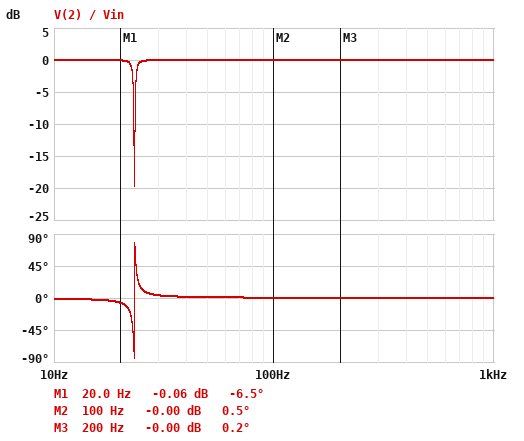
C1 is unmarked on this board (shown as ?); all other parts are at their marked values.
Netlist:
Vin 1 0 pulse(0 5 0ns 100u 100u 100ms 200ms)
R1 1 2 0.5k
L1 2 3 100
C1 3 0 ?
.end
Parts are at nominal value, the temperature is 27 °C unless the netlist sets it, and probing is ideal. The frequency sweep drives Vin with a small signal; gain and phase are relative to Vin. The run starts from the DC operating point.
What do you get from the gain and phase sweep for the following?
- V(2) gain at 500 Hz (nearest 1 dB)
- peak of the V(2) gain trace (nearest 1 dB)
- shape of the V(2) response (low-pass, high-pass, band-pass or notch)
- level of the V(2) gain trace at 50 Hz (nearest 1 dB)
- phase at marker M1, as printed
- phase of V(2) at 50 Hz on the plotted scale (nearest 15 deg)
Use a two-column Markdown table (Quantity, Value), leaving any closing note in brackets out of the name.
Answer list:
| Quantity | Value |
|---|---|
| V(2) gain at 500 Hz | 0 dB |
| peak of the V(2) gain trace | 0 dB |
| shape of the V(2) response | notch |
| level of the V(2) gain trace at 50 Hz | 0 dB |
| phase at marker M1, as printed | -6.5 deg |
| phase of V(2) at 50 Hz on the plotted scale | 0 deg |
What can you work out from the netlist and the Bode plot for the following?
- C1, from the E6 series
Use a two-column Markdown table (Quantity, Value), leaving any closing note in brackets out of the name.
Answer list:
| Quantity | Value |
|---|---|
| C1, from the E6 series | 470 nF |
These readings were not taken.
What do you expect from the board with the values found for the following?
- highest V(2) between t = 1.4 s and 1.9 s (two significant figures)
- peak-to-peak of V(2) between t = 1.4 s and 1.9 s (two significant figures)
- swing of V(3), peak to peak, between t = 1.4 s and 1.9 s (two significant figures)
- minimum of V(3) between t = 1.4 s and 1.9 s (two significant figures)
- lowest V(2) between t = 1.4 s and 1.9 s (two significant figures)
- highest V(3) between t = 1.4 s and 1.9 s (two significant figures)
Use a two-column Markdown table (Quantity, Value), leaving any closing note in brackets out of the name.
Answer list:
| Quantity | Value |
|---|---|
| highest V(2) between t = 1.4 s and 1.9 s | 5.2 V |
| peak-to-peak of V(2) between t = 1.4 s and 1.9 s | 5.3 V |
| swing of V(3), peak to peak, between t = 1.4 s and 1.9 s | 15 V |
| minimum of V(3) between t = 1.4 s and 1.9 s | -4.8 V |
| lowest V(2) between t = 1.4 s and 1.9 s | -160 mV |
| highest V(3) between t = 1.4 s and 1.9 s | 9.8 V |
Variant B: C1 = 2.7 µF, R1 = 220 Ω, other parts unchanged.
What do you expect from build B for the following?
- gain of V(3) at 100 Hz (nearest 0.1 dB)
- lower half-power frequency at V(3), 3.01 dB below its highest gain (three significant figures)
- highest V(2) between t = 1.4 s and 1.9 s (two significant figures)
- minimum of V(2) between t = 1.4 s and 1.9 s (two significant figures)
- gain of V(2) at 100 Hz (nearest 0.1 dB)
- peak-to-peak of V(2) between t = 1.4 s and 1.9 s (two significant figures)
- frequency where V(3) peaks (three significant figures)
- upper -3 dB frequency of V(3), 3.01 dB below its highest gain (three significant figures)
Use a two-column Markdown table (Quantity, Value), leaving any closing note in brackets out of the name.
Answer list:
| Quantity | Value |
|---|---|
| gain of V(3) at 100 Hz | -40.5 dB |
| lower half-power frequency at V(3), 3.01 dB below its highest gain | 9.51 Hz |
| highest V(2) between t = 1.4 s and 1.9 s | 5.1 V |
| minimum of V(2) between t = 1.4 s and 1.9 s | -100 mV |
| gain of V(2) at 100 Hz | 0 dB |
| peak-to-peak of V(2) between t = 1.4 s and 1.9 s | 5.2 V |
| frequency where V(3) peaks | 9.68 Hz |
| upper -3 dB frequency of V(3), 3.01 dB below its highest gain | 9.86 Hz |
